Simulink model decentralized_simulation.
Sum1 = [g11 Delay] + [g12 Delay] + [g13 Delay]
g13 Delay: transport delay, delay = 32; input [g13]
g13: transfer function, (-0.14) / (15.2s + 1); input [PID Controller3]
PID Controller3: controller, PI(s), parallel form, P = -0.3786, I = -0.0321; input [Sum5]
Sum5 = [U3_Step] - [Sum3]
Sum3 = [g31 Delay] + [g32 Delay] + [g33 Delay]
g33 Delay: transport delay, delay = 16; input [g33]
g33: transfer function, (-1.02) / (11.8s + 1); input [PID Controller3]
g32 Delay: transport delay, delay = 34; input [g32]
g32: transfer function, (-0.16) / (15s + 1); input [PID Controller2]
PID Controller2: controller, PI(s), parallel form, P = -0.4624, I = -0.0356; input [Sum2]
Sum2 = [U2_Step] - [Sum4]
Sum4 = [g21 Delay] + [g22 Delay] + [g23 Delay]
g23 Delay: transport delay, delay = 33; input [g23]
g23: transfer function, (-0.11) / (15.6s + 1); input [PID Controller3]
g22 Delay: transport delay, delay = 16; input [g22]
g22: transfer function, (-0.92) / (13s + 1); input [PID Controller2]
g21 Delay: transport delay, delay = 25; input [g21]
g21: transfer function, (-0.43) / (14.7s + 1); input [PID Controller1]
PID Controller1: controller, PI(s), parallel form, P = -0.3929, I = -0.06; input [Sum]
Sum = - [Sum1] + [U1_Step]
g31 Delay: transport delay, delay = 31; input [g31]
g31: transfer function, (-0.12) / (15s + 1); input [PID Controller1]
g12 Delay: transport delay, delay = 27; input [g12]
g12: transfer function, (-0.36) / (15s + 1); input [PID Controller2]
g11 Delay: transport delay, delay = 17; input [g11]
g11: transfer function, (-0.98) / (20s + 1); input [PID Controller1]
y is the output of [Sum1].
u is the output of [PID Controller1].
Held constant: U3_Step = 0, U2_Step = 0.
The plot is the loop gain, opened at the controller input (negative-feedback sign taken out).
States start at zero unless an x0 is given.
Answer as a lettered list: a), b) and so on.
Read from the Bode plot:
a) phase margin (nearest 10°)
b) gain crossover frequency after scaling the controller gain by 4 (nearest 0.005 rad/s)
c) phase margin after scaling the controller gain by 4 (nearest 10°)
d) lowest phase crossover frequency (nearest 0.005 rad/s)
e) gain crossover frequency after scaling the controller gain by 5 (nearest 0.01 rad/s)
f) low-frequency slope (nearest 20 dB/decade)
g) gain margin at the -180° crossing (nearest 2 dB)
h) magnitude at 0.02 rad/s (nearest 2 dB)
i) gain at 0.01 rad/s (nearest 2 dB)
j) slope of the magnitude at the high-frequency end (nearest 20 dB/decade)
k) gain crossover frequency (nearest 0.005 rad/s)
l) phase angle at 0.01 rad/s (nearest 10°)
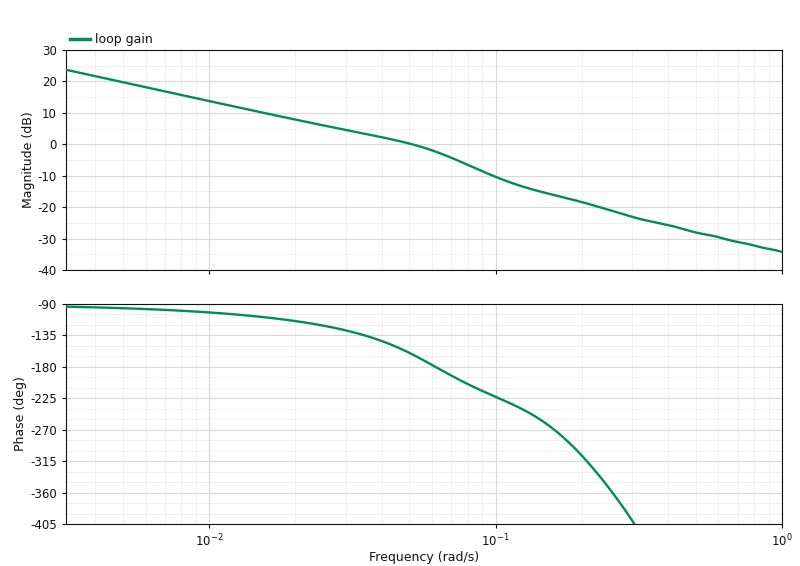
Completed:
a) 20°
b) 0.110 rad/s
c) -50°
d) 0.060 rad/s
e) 0.13 rad/s
f) -20 dB/decade
g) 2 dB
h) 8 dB
i) 14 dB
j) -20 dB/decade
k) 0.050 rad/s
l) -100°
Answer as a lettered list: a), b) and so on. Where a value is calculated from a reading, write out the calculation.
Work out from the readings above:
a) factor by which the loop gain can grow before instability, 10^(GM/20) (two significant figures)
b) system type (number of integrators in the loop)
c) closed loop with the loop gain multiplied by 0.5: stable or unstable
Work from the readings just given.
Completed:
a) 10^(2 / 20) = 1.3
b) 1
c) stable
